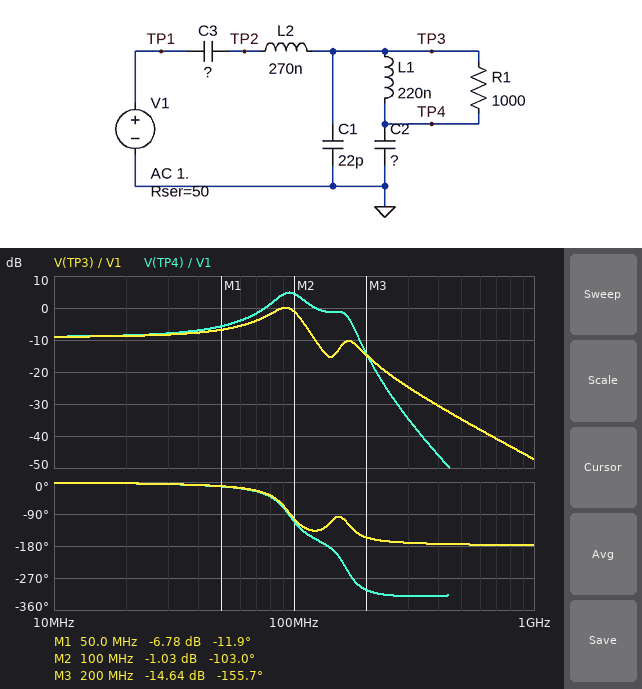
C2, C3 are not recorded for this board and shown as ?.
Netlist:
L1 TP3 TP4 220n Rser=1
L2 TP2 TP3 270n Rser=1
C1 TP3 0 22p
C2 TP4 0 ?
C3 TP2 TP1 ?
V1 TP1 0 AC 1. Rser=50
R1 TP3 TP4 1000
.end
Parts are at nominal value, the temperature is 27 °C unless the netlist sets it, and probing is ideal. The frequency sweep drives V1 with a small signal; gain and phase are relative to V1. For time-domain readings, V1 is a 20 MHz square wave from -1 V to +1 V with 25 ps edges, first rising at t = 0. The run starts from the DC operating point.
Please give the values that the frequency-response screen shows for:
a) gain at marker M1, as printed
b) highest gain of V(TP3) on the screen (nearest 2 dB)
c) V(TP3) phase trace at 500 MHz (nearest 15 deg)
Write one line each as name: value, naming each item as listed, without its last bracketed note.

gain at marker M1, as printed: -6.78 dB
highest gain of V(TP3) on the screen: 0 dB
V(TP3) phase trace at 500 MHz: -180 deg
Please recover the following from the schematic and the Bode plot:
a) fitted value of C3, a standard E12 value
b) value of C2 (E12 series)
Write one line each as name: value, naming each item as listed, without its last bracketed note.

fitted value of C3, a standard E12 value: 15 pF
value of C2: 5.6 pF
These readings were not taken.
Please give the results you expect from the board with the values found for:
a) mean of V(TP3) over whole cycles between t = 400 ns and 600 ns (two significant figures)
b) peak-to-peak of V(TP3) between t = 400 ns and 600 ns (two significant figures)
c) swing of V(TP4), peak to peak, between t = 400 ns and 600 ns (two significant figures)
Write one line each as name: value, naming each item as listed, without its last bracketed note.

mean of V(TP3) over whole cycles between t = 400 ns and 600 ns: 350 mV
peak-to-peak of V(TP3) between t = 400 ns and 600 ns: 1.4 V
swing of V(TP4), peak to peak, between t = 400 ns and 600 ns: 2.4 V
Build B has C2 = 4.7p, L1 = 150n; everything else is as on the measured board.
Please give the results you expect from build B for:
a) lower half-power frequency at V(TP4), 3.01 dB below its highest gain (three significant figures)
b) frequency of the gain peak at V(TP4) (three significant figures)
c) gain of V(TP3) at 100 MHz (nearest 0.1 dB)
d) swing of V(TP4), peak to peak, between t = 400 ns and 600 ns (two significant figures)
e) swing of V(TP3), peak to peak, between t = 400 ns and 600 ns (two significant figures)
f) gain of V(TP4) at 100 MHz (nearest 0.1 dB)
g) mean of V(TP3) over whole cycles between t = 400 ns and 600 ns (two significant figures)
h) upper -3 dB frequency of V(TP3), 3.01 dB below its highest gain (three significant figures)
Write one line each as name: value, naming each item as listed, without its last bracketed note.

lower half-power frequency at V(TP4), 3.01 dB below its highest gain: 81.6 MHz
frequency of the gain peak at V(TP4): 96.7 MHz
gain of V(TP3) at 100 MHz: 0.6 dB
swing of V(TP4), peak to peak, between t = 400 ns and 600 ns: 2.1 V
swing of V(TP3), peak to peak, between t = 400 ns and 600 ns: 1.6 V
gain of V(TP4) at 100 MHz: 3.4 dB
mean of V(TP3) over whole cycles between t = 400 ns and 600 ns: 360 mV
upper -3 dB frequency of V(TP3), 3.01 dB below its highest gain: 109 MHz
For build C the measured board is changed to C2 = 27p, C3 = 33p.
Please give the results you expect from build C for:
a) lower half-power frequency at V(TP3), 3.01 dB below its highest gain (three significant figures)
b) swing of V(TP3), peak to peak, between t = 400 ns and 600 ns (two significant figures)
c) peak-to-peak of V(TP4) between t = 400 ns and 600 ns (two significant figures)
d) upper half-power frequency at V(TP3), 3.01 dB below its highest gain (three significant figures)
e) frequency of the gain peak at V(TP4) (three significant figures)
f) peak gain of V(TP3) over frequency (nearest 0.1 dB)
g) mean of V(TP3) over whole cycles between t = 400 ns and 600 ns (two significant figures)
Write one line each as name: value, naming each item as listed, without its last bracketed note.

lower half-power frequency at V(TP3), 3.01 dB below its highest gain: 102 MHz
swing of V(TP3), peak to peak, between t = 400 ns and 600 ns: 1.6 V
peak-to-peak of V(TP4) between t = 400 ns and 600 ns: 2.6 V
upper half-power frequency at V(TP3), 3.01 dB below its highest gain: 125 MHz
frequency of the gain peak at V(TP4): 58.2 MHz
peak gain of V(TP3) over frequency: 3.2 dB
mean of V(TP3) over whole cycles between t = 400 ns and 600 ns: 400 mV
